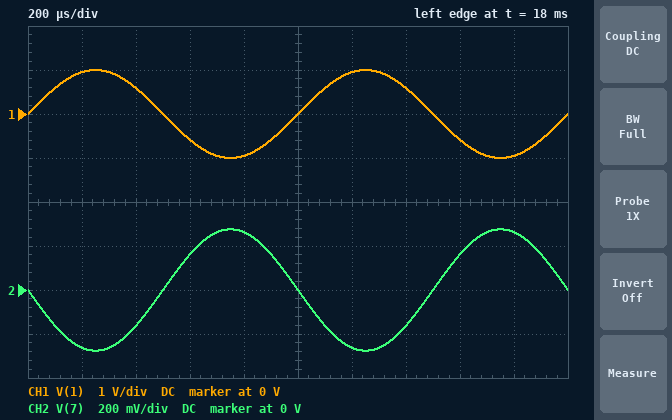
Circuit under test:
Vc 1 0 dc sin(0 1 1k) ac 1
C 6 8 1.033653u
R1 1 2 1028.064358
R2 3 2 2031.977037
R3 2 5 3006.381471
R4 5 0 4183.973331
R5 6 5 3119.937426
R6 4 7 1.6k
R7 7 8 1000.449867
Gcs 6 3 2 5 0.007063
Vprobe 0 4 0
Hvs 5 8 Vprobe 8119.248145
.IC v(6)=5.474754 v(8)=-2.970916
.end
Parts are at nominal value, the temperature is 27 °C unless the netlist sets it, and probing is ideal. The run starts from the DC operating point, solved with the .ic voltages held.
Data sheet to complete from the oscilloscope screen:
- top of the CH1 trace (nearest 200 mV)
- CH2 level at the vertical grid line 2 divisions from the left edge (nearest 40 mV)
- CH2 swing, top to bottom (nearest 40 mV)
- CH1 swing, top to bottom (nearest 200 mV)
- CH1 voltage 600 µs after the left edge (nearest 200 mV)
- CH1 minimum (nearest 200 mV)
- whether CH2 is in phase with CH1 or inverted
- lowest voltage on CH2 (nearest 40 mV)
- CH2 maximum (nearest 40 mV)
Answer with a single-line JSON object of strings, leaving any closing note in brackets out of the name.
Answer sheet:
{"top of the CH1 trace": "1.0 V", "CH2 level at the vertical grid line 2 divisions from the left edge": "-160 mV", "CH2 swing, top to bottom": "560 mV", "CH1 swing, top to bottom": "2.0 V", "CH1 voltage 600 µs after the left edge": "-600 mV", "CH1 minimum": "-1.0 V", "whether CH2 is in phase with CH1 or inverted": "inverted", "lowest voltage on CH2": "-280 mV", "CH2 maximum": "280 mV"}
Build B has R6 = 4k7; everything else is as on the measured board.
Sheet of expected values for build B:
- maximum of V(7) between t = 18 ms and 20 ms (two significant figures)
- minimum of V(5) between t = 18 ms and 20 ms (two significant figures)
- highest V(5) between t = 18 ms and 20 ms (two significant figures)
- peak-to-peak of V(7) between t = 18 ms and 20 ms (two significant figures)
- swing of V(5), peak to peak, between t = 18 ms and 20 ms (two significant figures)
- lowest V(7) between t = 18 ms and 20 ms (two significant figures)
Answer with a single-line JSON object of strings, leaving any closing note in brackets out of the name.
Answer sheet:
{"maximum of V(7) between t = 18 ms and 20 ms": "2.3 V", "minimum of V(5) between t = 18 ms and 20 ms": "-1.2 V", "highest V(5) between t = 18 ms and 20 ms": "1.2 V", "peak-to-peak of V(7) between t = 18 ms and 20 ms": "4.6 V", "swing of V(5), peak to peak, between t = 18 ms and 20 ms": "2.4 V", "lowest V(7) between t = 18 ms and 20 ms": "-2.3 V"}
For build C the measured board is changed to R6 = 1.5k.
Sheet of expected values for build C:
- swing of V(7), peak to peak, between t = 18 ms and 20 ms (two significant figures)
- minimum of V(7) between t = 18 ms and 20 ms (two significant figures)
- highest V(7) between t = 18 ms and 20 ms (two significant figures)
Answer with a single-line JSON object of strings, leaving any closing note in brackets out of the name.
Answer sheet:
{"swing of V(7), peak to peak, between t = 18 ms and 20 ms": "510 mV", "minimum of V(7) between t = 18 ms and 20 ms": "-250 mV", "highest V(7) between t = 18 ms and 20 ms": "250 mV"}
